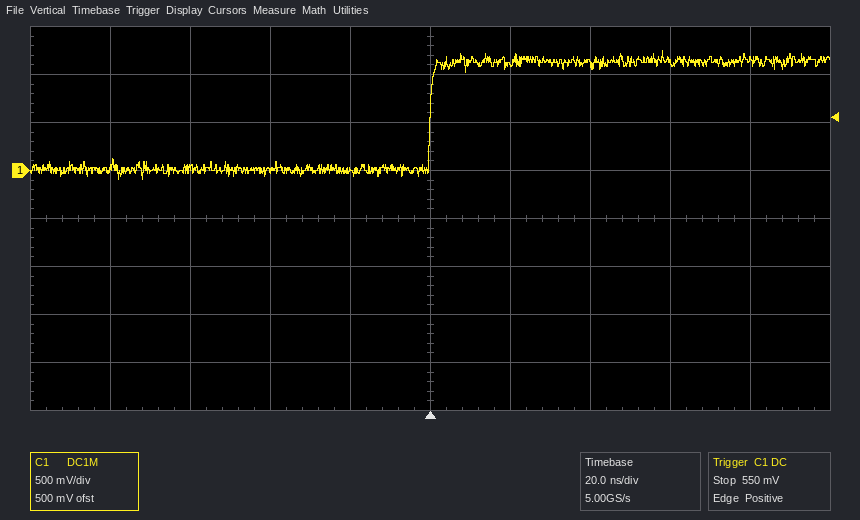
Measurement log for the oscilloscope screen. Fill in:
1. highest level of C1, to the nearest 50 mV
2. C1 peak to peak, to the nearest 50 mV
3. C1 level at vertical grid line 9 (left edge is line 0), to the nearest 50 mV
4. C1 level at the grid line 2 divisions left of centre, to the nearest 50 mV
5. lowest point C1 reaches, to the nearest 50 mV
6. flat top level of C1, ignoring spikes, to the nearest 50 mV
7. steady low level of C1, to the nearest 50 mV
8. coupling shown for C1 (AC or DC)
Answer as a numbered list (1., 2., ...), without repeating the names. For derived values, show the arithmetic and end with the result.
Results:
1. 1.25 V
2. 1.25 V − (-100 mV) = 1.35 V
3. 1.15 V
4. 0 mV
5. -100 mV
6. 1.15 V
7. 0 mV
8. DC
